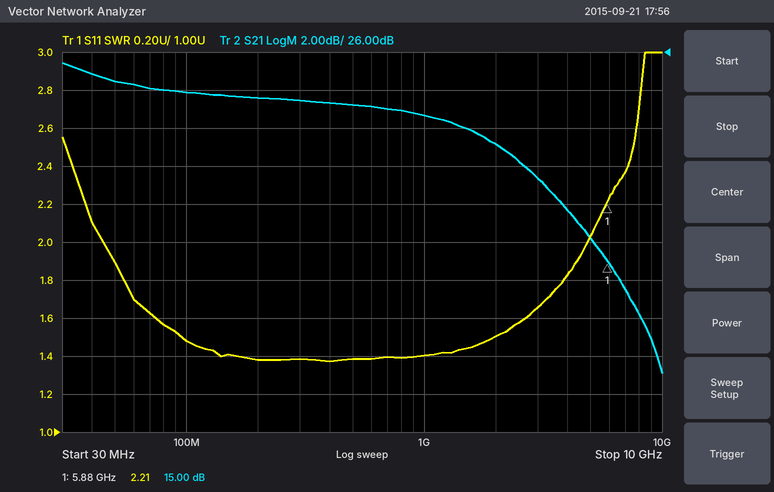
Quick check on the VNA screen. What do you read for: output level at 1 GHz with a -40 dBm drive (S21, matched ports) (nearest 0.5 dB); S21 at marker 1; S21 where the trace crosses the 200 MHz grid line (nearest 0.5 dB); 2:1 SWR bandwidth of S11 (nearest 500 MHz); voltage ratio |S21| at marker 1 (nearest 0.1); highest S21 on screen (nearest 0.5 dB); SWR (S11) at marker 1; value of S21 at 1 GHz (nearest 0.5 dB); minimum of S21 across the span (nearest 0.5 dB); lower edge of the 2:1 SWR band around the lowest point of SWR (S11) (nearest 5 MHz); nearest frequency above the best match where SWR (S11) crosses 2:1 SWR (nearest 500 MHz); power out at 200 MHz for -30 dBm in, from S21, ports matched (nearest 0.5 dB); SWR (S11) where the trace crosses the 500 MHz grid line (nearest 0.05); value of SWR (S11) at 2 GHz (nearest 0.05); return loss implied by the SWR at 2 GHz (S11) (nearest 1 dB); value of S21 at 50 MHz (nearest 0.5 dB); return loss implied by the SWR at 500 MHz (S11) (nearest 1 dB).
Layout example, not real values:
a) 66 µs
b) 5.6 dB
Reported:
a) -17.5 dBm
b) 15.00 dB
c) 23.5 dB
d) 5.0 GHz
e) 5.6
f) 25.5 dB
g) 2.21
h) 22.5 dB
i) 9.0 dB
j) 45 MHz
k) 5.0 GHz
l) -6.5 dBm
m) 1.40
n) 1.50
o) 14 dB
p) 24.5 dB
q) 16 dB
